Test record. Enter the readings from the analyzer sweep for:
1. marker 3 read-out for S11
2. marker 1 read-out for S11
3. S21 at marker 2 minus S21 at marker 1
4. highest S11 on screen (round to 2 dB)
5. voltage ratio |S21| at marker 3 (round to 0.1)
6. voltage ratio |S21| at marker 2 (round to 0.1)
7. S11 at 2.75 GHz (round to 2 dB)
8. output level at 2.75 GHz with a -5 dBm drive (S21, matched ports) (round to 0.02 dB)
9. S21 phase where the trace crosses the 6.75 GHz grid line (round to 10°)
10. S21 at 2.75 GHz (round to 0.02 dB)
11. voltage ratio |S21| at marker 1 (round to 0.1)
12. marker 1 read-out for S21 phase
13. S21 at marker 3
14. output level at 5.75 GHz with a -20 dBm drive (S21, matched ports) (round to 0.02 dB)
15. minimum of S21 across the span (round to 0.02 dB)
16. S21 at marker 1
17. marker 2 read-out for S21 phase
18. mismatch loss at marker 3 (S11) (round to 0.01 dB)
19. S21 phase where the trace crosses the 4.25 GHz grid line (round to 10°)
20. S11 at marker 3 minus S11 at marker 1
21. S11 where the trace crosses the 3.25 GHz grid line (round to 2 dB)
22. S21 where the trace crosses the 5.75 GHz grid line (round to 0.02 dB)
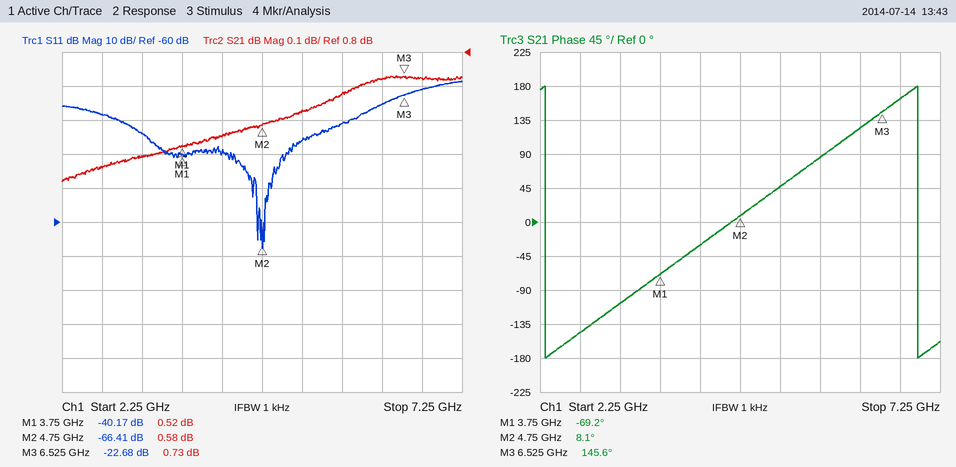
-22.68 dB
-40.17 dB
0.06 dB
-18 dB
1.1
1.1
-28 dB
-4.54 dBm
160°
0.46 dB
1.1
-69.2°
0.73 dB
-19.32 dBm
0.42 dB
0.52 dB
8.1°
0.02 dB
-30°
17.49 dB
-34 dB
0.68 dB
